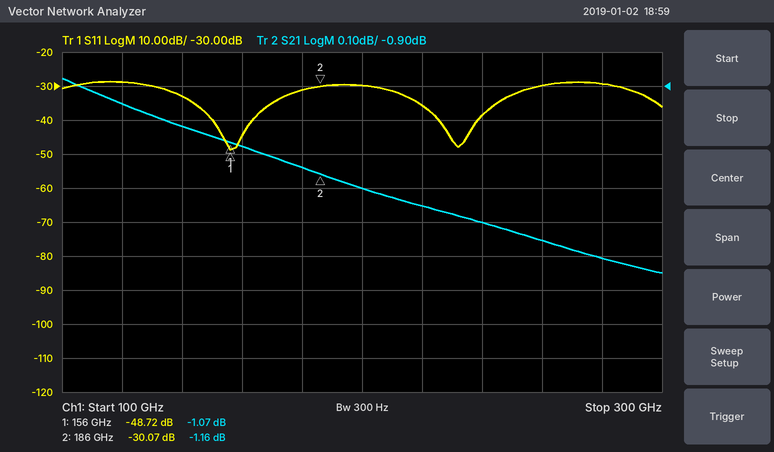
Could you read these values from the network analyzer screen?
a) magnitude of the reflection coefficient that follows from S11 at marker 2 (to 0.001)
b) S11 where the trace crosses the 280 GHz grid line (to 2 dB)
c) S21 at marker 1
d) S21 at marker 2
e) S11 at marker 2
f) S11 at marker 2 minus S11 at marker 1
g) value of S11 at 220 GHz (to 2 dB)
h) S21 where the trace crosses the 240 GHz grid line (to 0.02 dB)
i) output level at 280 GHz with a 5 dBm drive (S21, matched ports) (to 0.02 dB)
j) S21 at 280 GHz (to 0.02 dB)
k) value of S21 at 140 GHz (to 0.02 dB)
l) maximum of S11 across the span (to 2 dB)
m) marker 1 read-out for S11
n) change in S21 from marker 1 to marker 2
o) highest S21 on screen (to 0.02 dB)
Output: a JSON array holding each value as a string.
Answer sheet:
["0.031", "-30 dB", "-1.07 dB", "-1.16 dB", "-30.07 dB", "18.65 dB", "-36 dB", "-1.30 dB", "3.60 dBm", "-1.40 dB", "-1.02 dB", "-28 dB", "-48.72 dB", "-0.09 dB", "-0.88 dB"]
